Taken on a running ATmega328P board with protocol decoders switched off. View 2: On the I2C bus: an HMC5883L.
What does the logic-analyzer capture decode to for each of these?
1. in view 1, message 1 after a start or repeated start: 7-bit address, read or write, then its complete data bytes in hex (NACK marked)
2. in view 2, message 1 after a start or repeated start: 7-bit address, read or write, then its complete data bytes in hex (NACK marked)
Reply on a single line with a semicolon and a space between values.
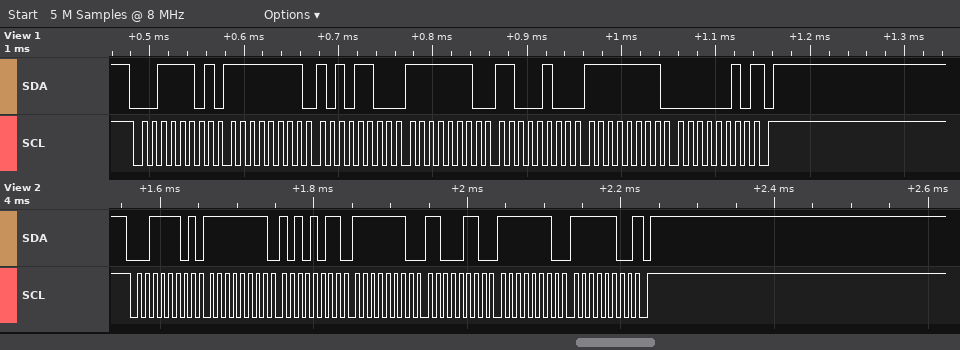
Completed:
0x1E read: FF AC FE C4 FF 02 NACK; 0x1E read: FF AB FE C6 FE FC NACK
